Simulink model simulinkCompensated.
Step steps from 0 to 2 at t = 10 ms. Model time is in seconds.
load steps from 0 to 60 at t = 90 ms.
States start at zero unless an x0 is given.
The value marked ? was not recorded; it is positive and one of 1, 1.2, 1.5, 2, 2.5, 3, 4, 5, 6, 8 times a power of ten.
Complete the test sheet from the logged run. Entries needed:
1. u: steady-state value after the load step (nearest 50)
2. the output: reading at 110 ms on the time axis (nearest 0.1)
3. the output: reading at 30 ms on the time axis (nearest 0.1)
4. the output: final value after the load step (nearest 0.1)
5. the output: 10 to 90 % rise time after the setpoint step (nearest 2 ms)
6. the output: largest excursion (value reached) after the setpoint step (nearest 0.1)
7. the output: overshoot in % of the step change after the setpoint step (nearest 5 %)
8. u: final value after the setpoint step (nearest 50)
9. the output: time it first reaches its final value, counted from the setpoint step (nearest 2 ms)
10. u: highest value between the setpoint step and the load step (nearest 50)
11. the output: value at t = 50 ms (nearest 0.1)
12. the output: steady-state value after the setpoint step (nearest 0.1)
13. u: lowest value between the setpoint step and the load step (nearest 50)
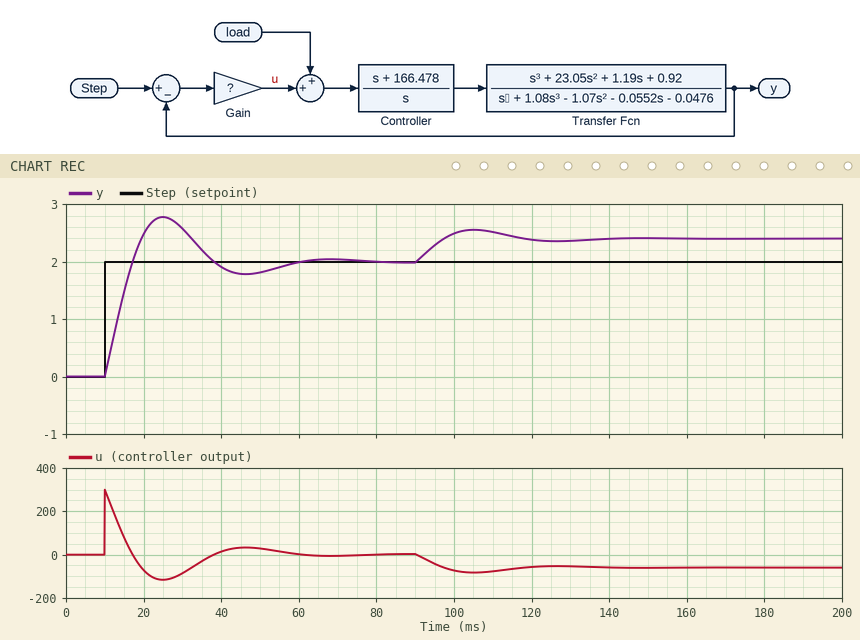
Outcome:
-50
2.5
2.6
2.4
6 ms
2.8
40 %
0
8 ms
300
1.8
2.0
-100
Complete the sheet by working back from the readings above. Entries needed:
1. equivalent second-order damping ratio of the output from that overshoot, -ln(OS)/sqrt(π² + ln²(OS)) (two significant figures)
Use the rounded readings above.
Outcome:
0.28
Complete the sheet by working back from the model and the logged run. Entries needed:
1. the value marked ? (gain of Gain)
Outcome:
150
